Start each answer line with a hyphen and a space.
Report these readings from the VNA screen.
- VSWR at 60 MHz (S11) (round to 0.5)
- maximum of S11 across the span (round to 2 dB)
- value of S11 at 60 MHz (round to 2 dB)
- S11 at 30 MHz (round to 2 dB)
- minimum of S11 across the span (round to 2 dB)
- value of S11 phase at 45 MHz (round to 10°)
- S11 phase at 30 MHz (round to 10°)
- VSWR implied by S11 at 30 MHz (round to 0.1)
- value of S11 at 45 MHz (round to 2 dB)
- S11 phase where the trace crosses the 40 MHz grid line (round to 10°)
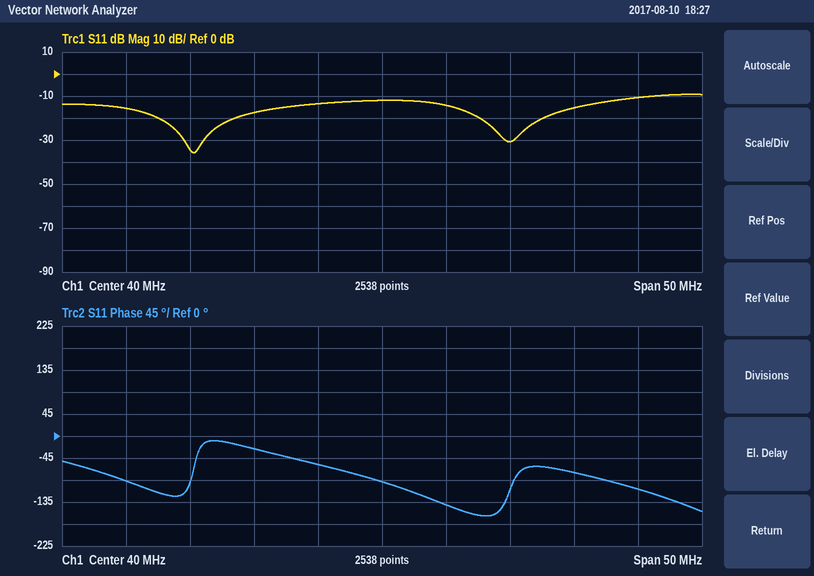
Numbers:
- 2.0
- -10 dB
- -10 dB
- -18 dB
- -36 dB
- -140°
- -30°
- 1.3
- -14 dB
- -90°
